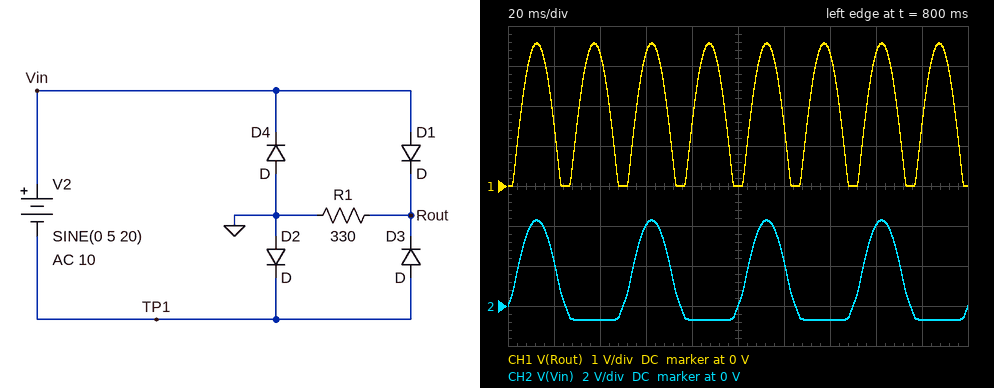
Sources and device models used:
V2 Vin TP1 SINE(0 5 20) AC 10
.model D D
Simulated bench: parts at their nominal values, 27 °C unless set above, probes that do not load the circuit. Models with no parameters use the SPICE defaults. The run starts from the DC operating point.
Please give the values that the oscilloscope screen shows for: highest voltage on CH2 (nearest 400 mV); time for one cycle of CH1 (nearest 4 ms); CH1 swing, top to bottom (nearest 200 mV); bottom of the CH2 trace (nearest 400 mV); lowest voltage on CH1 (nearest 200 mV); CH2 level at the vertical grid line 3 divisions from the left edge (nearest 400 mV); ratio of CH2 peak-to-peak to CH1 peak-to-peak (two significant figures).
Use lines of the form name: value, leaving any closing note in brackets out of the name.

highest voltage on CH2: 4.4 V
time for one cycle of CH1: 24 ms
CH1 swing, top to bottom: 3.6 V
bottom of the CH2 trace: -800 mV
lowest voltage on CH1: 0 V
CH2 level at the vertical grid line 3 divisions from the left edge: 4.0 V
ratio of CH2 peak-to-peak to CH1 peak-to-peak: 1.4
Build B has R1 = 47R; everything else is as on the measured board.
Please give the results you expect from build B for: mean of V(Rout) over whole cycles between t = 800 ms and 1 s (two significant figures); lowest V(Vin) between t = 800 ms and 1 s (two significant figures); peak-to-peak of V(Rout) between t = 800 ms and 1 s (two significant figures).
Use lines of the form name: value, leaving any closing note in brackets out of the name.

mean of V(Rout) over whole cycles between t = 800 ms and 1 s: 1.8 V
lowest V(Vin) between t = 800 ms and 1 s: -770 mV
peak-to-peak of V(Rout) between t = 800 ms and 1 s: 3.5 V
